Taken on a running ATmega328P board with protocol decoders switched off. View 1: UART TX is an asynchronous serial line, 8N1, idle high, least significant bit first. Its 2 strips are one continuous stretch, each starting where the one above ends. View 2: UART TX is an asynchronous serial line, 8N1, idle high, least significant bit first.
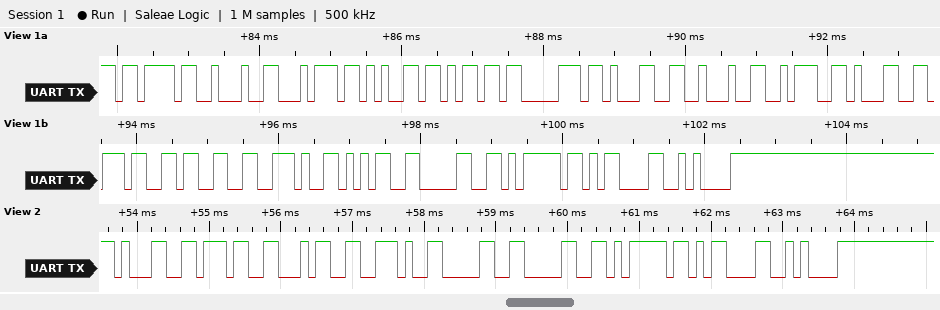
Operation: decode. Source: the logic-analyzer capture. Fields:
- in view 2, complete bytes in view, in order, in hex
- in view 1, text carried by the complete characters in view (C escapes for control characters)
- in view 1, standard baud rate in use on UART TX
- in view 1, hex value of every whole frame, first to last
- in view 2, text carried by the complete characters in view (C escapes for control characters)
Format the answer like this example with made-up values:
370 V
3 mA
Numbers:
0x31 0x37 0x34 0x2E 0x30 0x30 0x7D 0x0D 0x0A
"{\"temp1\":173.50}\r\n"
9600 baud
7B 22 74 65 6D 70 31 22 3A 31 37 33 2E 35 30 7D 0D 0A
"174.00}\r\n"
